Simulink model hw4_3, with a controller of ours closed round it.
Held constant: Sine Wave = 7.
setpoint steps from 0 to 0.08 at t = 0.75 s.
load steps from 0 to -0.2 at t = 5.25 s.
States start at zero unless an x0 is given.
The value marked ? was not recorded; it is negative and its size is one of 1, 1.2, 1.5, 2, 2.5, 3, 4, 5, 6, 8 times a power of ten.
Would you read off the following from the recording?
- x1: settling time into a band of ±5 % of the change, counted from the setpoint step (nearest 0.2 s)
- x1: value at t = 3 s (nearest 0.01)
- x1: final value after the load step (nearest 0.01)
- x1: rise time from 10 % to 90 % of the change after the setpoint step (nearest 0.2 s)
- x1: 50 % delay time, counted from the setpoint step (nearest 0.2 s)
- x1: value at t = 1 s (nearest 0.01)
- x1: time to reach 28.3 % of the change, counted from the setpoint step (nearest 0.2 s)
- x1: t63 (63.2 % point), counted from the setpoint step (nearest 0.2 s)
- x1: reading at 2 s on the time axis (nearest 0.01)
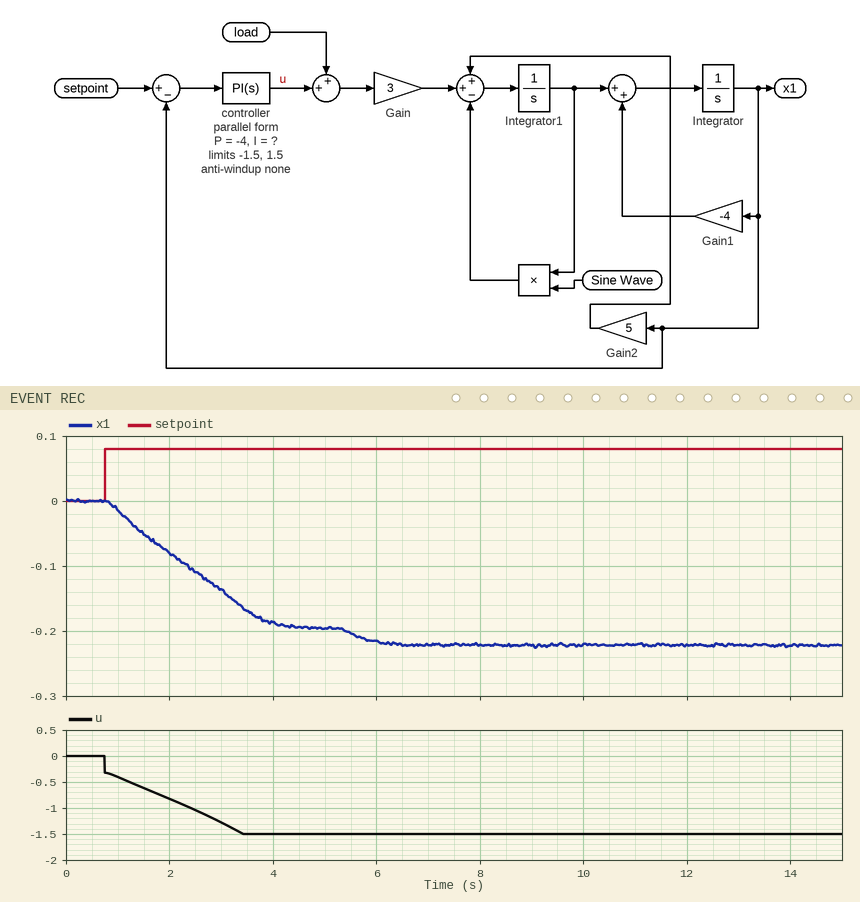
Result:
3.2 s
-0.14
-0.22
2.6 s
1.6 s
-0.01
0.8 s
2.0 s
-0.08
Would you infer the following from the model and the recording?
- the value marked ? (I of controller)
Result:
-1.2
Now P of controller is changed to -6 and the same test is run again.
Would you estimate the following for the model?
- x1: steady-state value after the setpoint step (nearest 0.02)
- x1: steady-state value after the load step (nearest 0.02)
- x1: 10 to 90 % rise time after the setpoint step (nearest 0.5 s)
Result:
-0.20
-0.22
1.5 s
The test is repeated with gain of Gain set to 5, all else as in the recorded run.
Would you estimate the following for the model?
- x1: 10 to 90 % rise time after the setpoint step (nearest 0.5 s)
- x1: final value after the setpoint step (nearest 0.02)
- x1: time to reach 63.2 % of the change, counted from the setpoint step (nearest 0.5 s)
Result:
1.5 s
-0.32
1.5 s
